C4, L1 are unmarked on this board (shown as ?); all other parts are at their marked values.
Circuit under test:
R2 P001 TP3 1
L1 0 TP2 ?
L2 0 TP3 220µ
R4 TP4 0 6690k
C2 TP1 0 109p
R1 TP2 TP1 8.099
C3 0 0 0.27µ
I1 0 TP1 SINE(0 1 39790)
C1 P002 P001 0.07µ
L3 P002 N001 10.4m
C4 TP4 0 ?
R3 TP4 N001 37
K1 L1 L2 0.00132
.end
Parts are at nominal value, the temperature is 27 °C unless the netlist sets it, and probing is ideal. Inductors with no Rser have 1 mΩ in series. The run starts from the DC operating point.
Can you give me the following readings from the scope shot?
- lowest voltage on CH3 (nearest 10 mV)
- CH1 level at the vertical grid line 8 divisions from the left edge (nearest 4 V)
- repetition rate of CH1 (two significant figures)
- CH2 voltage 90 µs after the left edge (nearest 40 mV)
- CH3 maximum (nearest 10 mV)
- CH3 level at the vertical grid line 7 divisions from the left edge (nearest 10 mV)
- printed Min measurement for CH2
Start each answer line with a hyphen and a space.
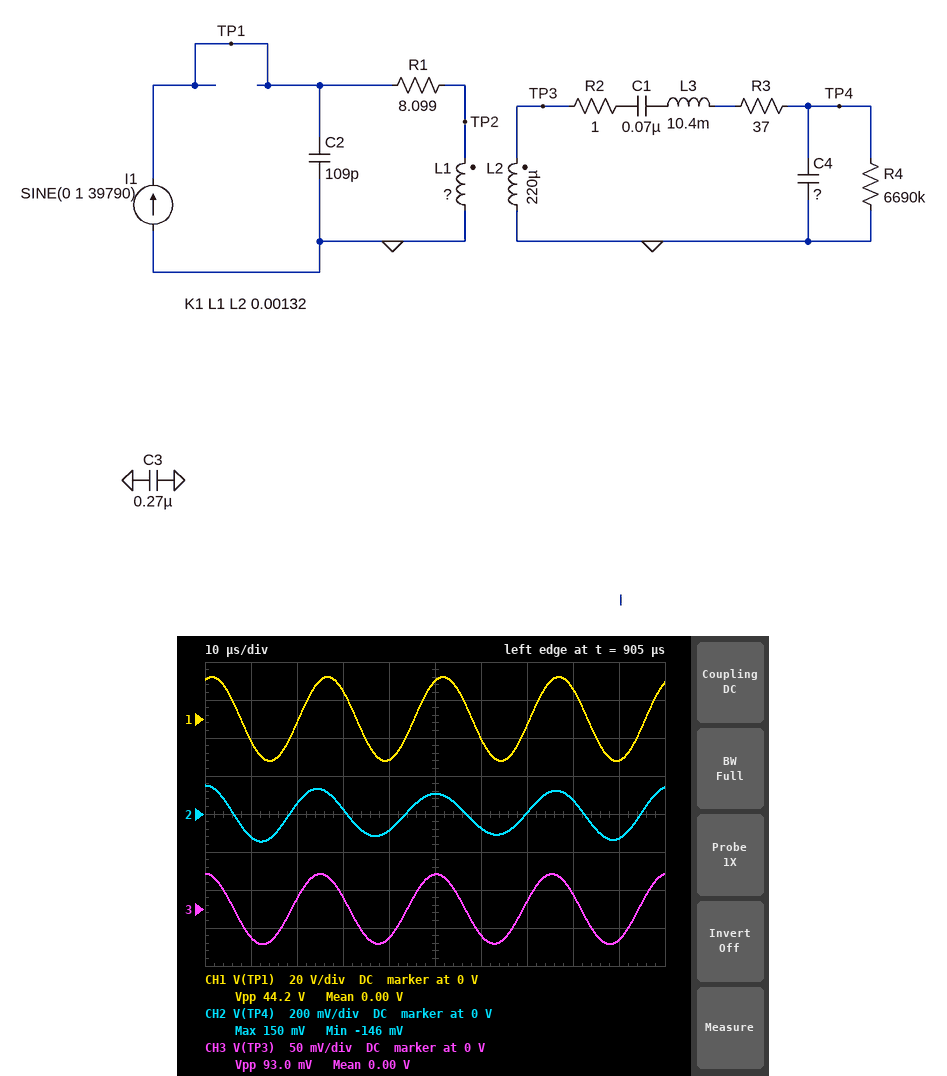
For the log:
- -50 mV
- 16 V
- 40 kHz
- -120 mV
- 50 mV
- 10 mV
- -146 mV
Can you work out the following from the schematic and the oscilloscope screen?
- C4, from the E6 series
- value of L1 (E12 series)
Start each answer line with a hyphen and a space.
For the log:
- 1 nF
- 82 µH
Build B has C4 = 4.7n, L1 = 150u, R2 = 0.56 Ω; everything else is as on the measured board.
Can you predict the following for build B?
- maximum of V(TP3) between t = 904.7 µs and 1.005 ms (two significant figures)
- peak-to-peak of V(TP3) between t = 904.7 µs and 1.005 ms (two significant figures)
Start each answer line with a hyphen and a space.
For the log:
- 58 mV
- 120 mV
